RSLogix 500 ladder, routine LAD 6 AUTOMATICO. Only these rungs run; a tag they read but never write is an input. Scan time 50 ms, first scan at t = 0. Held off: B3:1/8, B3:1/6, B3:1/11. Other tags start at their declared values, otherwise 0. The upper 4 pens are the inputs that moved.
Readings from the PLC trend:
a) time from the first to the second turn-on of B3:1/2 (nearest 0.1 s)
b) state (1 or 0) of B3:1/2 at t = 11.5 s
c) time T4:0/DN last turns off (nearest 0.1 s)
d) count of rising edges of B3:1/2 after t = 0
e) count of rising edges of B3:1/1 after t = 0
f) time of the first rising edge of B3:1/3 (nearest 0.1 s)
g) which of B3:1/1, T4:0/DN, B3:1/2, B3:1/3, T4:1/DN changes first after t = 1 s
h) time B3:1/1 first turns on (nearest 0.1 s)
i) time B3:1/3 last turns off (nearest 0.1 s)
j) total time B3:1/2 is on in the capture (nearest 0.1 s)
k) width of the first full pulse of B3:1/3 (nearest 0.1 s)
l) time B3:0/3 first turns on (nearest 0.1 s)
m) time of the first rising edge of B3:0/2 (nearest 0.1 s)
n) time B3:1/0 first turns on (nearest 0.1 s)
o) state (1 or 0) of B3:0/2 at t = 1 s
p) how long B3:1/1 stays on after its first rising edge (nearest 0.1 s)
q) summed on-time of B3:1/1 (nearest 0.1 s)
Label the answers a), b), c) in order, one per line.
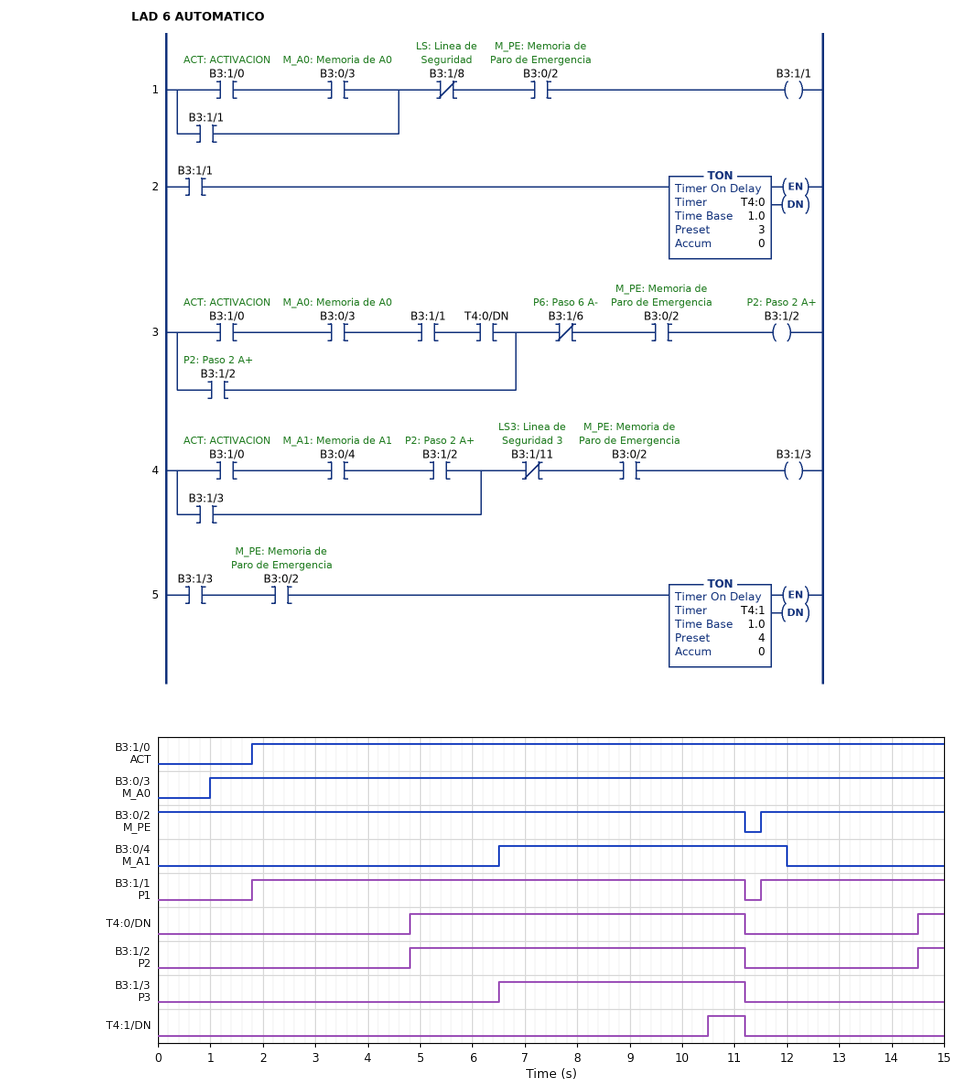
a) 9.7 s
b) 0
c) 11.2 s
d) 2
e) 2
f) 6.5 s
g) B3:1/1
h) 1.8 s
i) 11.2 s
j) 6.9 s
k) 4.7 s
l) 1.0 s
m) 11.5 s
n) 1.8 s
o) 1
p) 9.4 s
q) 12.9 s
